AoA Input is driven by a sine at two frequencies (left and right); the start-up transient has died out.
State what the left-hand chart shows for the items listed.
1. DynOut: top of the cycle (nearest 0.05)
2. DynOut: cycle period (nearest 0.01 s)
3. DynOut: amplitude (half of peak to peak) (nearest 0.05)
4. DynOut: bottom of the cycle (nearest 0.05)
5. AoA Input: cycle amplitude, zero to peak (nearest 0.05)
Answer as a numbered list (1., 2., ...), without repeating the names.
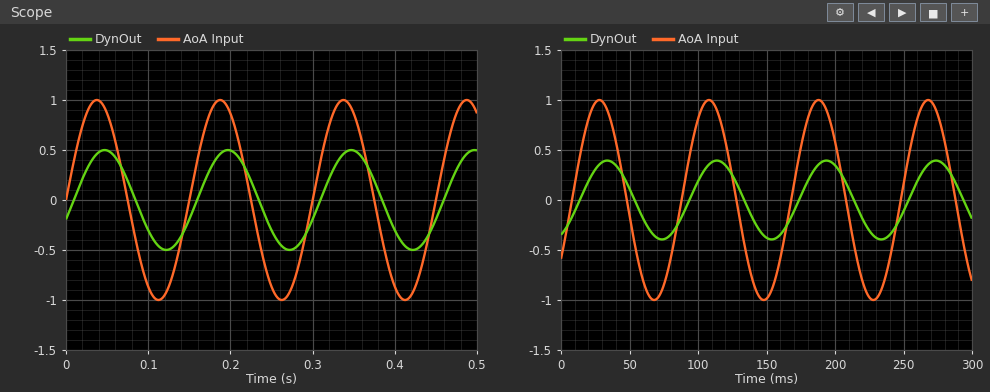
1. 0.50
2. 0.15 s
3. 0.50
4. -0.50
5. 1.00
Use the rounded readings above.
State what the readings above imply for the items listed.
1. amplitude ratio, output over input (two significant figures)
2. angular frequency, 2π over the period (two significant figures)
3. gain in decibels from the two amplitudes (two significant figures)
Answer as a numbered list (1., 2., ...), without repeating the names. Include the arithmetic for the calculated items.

1. 0.5 / 1 = 0.50
2. 2π / 0.15 = 42 rad/s
3. 20 log10(0.5 / 1) = -6.0 dB
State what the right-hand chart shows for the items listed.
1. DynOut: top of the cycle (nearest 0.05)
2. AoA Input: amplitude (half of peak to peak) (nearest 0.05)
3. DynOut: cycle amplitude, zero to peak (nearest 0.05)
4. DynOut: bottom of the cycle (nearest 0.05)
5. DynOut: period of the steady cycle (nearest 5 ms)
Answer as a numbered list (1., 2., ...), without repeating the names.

1. 0.40
2. 1.00
3. 0.40
4. -0.40
5. 80 ms
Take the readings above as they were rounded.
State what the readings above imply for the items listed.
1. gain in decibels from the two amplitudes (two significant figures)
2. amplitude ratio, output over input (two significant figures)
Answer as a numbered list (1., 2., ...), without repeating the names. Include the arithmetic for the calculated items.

1. 20 log10(0.4 / 1) = -8.0 dB
2. 0.4 / 1 = 0.40
